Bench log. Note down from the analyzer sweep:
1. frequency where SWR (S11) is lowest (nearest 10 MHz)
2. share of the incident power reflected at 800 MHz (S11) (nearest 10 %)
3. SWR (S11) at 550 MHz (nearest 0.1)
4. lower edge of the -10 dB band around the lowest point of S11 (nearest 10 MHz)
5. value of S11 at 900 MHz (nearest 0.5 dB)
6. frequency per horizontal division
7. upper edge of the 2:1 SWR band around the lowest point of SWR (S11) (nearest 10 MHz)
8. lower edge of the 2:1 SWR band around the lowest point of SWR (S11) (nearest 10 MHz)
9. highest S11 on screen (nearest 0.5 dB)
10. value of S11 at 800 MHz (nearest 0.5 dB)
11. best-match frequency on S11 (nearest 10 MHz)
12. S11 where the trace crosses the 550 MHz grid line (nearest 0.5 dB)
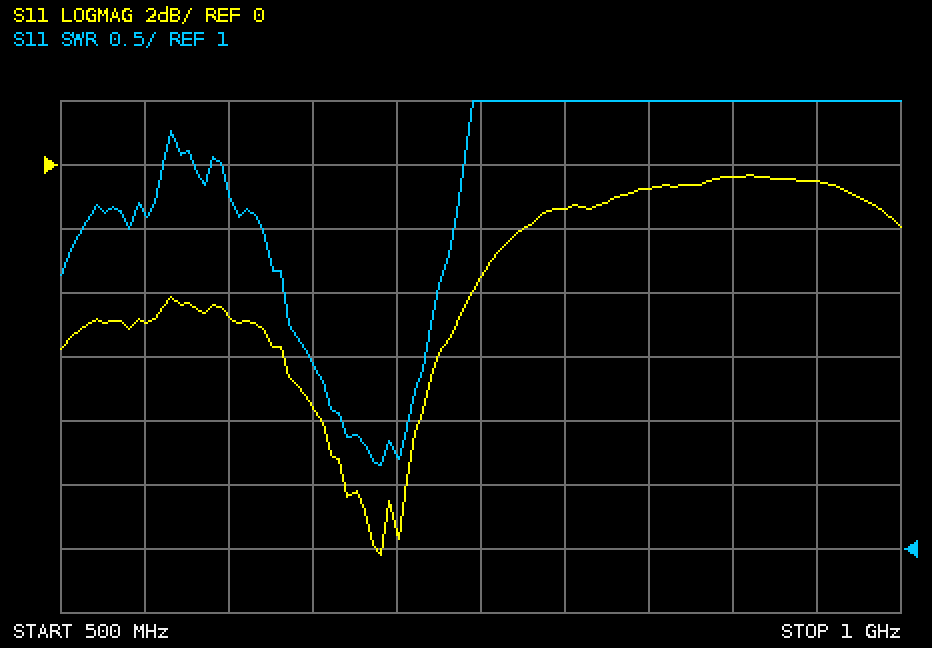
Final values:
690 MHz
70 %
3.6
670 MHz
-0.5 dB
50 MHz
710 MHz
670 MHz
-0.5 dB
-1.5 dB
690 MHz
-5.0 dB
